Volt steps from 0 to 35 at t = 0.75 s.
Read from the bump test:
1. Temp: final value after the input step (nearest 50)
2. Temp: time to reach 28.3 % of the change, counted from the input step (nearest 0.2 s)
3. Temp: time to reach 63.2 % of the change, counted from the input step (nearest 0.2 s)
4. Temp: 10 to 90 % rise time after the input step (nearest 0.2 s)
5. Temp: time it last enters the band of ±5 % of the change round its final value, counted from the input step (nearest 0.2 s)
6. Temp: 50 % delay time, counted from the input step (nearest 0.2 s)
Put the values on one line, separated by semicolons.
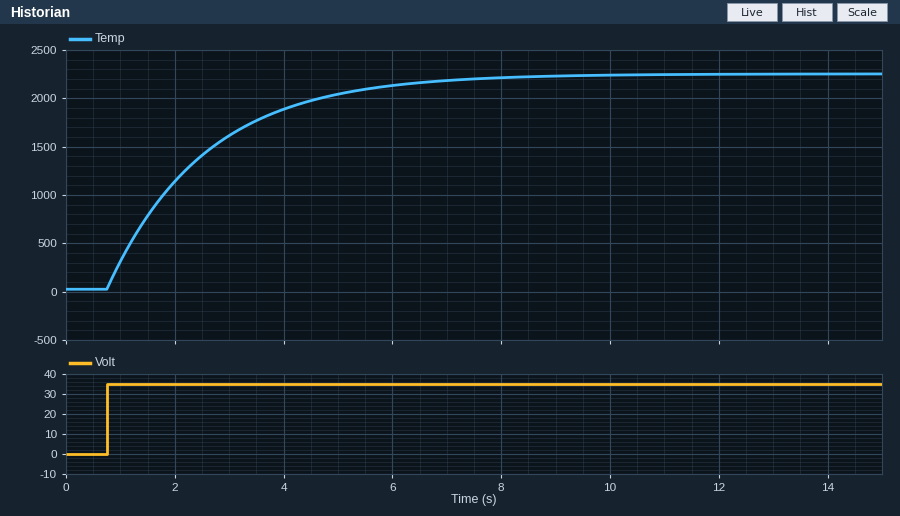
2250; 0.6 s; 1.8 s; 4.0 s; 5.4 s; 1.2 s
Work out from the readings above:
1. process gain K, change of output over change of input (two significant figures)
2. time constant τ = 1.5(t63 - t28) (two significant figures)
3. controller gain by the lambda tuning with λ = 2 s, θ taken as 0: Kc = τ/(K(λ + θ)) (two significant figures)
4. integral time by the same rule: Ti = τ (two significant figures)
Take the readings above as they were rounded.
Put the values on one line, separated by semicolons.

64; 1.8 s; 0.014; 1.8 s
